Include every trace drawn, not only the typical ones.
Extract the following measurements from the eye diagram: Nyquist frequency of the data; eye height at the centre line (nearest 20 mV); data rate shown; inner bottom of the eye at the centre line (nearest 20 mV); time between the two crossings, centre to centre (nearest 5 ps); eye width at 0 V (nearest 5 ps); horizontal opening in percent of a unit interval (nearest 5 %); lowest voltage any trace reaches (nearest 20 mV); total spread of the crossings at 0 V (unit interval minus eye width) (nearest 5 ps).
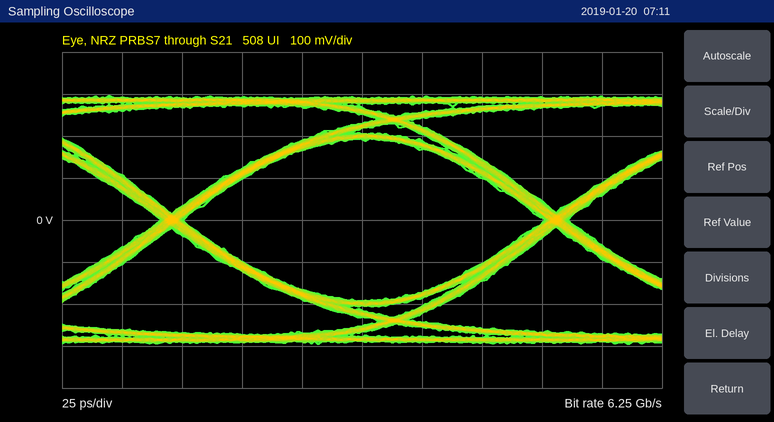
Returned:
3.125 GHz
380 mV
6.25 Gb/s
-200 mV
160 ps
150 ps
95 %
-300 mV
10 ps
